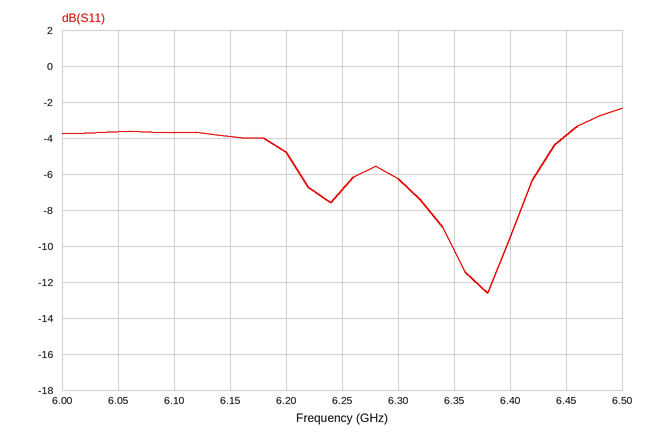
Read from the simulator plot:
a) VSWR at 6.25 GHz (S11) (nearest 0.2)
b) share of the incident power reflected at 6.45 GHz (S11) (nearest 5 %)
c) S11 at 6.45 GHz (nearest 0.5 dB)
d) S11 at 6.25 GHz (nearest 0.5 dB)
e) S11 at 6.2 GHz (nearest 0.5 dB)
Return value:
2.6
40 %
-4.0 dB
-7.0 dB
-5.0 dB
